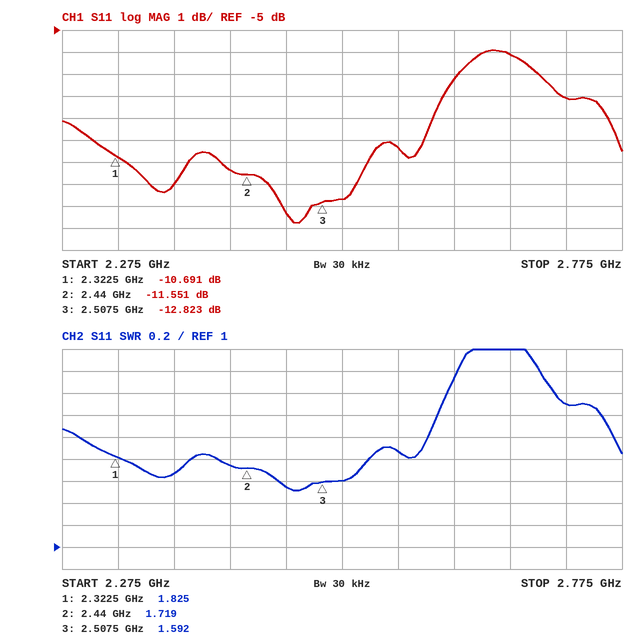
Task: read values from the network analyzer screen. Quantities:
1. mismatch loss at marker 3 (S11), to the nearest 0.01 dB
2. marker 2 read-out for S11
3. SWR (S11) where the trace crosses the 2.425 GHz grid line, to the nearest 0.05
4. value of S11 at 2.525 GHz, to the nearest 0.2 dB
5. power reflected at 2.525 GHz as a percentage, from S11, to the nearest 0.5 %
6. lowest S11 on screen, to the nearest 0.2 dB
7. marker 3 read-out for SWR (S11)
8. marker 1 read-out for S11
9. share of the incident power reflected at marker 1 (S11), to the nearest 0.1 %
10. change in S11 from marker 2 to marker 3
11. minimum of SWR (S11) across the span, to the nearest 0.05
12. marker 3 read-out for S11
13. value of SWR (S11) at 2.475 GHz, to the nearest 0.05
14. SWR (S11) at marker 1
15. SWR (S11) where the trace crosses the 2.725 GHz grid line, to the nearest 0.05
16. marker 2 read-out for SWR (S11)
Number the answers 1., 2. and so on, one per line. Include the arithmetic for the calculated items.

1. −10 log10(1 − 10^(-12.823/10)) ≈ 0.23 dB
2. -11.551 dB
3. 1.75
4. -12.6 dB
5. 10^(-12.6/10) ≈ 5.5 %
6. -13.8 dB
7. 1.592
8. -10.691 dB
9. 10^(-10.691/10) ≈ 8.5 %
10. -12.823 − (-11.551) = -1.272 dB
11. 1.50
12. -12.823 dB
13. 1.55
14. 1.825
15. 2.30
16. 1.719
